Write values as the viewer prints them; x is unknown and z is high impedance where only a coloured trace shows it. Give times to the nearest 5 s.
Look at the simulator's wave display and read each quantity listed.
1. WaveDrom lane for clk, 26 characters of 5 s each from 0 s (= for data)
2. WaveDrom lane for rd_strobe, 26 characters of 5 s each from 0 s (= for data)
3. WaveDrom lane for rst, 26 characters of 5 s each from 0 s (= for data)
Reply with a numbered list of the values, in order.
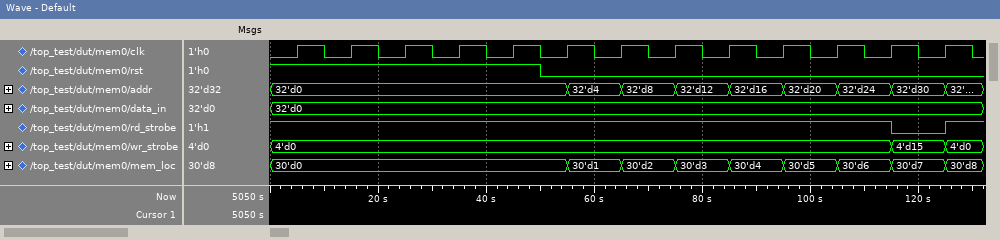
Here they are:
1. {name: 'clk', wave: '01010101010101010101010101'}
2. {name: 'rd_strobe', wave: '1......................0.1'}
3. {name: 'rst', wave: '1.........0...............'}
